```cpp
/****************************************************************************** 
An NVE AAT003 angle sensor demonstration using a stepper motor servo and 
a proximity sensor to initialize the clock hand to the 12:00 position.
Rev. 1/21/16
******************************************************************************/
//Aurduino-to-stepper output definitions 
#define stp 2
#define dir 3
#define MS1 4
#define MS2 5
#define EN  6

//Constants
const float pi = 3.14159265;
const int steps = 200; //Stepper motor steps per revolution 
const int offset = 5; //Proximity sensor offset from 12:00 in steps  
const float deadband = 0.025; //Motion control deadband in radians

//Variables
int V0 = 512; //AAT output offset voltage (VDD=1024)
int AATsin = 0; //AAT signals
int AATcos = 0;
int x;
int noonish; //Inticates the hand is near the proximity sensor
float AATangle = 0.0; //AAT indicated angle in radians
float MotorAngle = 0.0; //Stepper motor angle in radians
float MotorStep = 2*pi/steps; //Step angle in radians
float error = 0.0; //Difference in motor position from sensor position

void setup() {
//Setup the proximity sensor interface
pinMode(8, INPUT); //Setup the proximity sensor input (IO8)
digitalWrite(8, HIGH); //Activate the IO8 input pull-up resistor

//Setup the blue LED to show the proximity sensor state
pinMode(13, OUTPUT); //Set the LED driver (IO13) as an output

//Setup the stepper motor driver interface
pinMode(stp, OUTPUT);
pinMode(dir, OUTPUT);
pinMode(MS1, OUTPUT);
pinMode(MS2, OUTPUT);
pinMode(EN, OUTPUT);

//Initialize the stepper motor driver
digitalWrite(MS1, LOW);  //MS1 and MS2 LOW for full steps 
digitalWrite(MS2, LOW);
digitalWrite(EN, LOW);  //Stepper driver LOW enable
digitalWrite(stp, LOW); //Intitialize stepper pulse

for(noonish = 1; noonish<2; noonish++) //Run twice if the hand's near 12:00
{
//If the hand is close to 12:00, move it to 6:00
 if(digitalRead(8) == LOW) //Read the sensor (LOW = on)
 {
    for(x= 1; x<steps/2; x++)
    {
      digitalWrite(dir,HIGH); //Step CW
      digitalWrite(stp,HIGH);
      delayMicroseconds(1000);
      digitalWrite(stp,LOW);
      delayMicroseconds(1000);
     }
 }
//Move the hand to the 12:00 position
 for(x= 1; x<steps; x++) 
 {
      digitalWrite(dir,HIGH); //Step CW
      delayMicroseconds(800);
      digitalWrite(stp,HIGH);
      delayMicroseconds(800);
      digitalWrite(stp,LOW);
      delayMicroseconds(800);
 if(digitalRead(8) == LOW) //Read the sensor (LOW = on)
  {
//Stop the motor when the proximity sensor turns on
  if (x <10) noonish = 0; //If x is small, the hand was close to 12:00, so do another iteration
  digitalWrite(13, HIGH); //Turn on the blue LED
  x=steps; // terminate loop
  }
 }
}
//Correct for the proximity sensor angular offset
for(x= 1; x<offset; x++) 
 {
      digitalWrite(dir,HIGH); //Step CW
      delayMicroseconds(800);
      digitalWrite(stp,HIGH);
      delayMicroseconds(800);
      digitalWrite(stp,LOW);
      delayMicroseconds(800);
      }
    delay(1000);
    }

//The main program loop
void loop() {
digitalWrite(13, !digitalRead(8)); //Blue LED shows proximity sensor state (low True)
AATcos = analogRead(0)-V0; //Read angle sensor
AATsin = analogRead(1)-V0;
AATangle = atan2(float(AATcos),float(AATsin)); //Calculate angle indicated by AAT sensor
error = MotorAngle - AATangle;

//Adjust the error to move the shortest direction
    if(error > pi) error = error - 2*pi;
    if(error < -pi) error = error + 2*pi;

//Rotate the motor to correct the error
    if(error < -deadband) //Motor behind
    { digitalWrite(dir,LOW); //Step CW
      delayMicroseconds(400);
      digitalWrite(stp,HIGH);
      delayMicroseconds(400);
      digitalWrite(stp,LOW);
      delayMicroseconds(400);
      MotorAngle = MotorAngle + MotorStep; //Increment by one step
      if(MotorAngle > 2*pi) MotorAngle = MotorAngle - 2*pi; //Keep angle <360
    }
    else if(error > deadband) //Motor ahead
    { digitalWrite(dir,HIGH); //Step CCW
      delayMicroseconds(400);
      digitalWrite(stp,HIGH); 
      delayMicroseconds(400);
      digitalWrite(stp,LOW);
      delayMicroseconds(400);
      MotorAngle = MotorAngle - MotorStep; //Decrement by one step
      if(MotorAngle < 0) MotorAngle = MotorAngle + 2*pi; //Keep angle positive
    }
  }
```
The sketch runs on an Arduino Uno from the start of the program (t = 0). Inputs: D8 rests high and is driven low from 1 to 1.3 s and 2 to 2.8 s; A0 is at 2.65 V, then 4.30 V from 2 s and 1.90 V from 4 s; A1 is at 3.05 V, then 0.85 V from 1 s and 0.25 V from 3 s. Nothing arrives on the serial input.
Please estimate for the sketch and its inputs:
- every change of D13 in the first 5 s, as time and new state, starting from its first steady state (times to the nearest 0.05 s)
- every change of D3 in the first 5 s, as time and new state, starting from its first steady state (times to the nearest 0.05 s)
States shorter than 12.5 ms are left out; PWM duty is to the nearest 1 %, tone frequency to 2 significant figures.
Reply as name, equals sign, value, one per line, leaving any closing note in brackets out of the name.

every change of D13 in the first 5 s, as time and new state, starting from its first steady state = 0 s low; 2 s high; 2.8 s low
every change of D3 in the first 5 s, as time and new state, starting from its first steady state = 0 s high; 1.5 s low; 2 s high; 3 s low
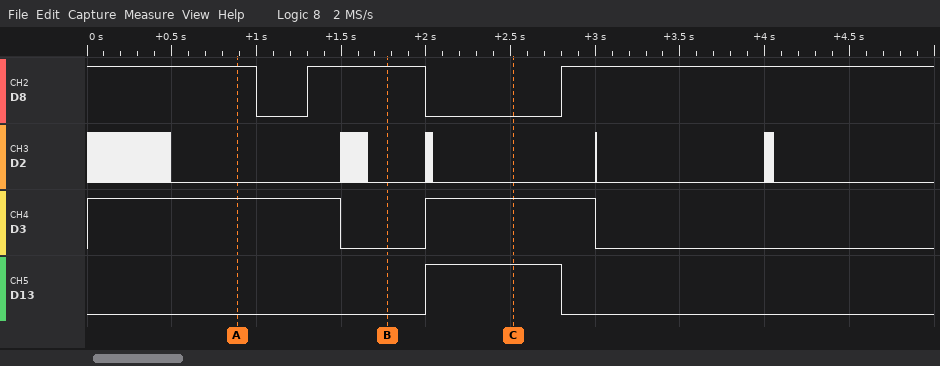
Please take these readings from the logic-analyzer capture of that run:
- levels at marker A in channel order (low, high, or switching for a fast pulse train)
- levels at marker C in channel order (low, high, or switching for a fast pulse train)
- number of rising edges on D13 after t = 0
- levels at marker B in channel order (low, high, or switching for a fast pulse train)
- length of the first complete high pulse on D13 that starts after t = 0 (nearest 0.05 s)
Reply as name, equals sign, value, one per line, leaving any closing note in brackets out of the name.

levels at marker A in channel order = D8 high, D2 low, D3 high, D13 low
levels at marker C in channel order = D8 low, D2 low, D3 high, D13 high
number of rising edges on D13 after t = 0 = 1
levels at marker B in channel order = D8 high, D2 low, D3 low, D13 low
length of the first complete high pulse on D13 that starts after t = 0 = 0.80 s
